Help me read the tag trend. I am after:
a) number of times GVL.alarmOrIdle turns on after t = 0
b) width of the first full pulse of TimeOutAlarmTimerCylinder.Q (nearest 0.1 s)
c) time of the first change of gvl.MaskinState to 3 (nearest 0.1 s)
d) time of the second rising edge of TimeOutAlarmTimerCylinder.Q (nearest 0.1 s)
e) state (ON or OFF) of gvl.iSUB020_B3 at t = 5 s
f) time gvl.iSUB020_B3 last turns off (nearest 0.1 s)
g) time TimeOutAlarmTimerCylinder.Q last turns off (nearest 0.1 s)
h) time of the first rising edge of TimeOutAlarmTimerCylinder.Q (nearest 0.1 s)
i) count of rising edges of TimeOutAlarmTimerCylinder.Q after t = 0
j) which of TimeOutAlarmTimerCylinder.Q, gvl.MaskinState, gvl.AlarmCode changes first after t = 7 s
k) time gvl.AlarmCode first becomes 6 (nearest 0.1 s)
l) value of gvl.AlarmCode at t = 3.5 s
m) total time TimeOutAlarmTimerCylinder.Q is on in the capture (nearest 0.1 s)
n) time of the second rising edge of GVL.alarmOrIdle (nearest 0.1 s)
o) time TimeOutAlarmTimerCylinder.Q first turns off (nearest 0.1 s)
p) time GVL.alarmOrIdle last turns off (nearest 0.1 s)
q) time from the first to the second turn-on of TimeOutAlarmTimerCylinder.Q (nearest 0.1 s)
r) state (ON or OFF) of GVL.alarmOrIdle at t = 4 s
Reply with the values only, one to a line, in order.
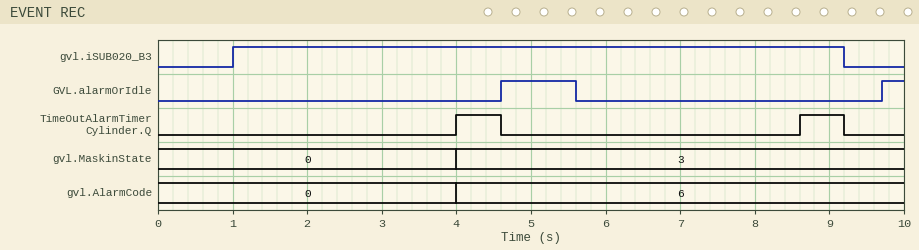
2
0.6 s
4.0 s
8.6 s
ON
9.2 s
9.2 s
4.0 s
2
TimeOutAlarmTimerCylinder.Q
4.0 s
0
1.2 s
9.7 s
4.6 s
5.6 s
4.6 s
OFF
